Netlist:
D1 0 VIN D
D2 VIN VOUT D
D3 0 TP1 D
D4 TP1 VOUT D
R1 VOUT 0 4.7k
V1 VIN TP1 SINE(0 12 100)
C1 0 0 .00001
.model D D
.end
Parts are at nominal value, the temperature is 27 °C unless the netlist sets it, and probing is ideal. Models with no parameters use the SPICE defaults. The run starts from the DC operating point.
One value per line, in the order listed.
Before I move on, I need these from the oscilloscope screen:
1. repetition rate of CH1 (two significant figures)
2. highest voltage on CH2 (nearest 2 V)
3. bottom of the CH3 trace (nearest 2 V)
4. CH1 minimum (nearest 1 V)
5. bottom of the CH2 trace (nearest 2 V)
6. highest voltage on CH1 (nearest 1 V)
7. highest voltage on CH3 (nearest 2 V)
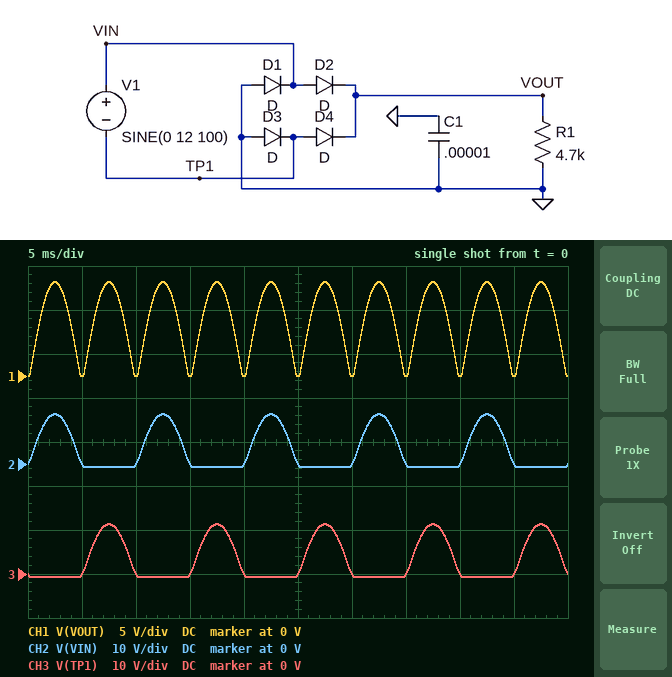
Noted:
200 Hz
12 V
0 V
0 V
0 V
11 V
12 V
